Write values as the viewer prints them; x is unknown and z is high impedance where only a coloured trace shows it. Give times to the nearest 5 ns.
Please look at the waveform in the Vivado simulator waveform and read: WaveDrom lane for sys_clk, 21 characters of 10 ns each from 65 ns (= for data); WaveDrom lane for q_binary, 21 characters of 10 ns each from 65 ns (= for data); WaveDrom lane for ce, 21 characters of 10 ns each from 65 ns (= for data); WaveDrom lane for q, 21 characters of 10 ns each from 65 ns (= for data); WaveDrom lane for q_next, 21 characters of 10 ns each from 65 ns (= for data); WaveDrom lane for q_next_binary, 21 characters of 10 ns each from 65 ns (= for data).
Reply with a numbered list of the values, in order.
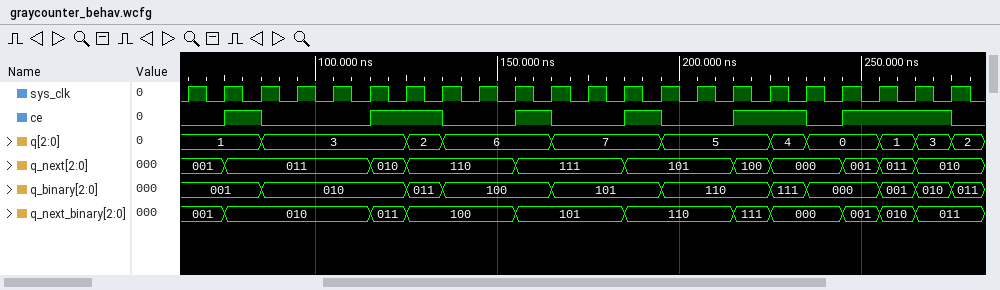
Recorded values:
1. {name: 'sys_clk', wave: 'p....................'}
2. {name: 'q_binary', wave: '=.=...==..=..=..==.==', data: '001 010 011 100 101 110 111 000 001 010'}
3. {name: 'ce', wave: '010..1.0.10.10.1.01..'}
4. {name: 'q', wave: '=.=...==..=..=..==.==', data: '1 3 2 6 7 5 4 0 1 3'}
5. {name: 'q_next', wave: '==...==..=..=..==.===', data: '001 011 010 110 111 101 100 000 001 011 010'}
6. {name: 'q_next_binary', wave: '==...==..=..=..==.===', data: '001 010 011 100 101 110 111 000 001 010 011'}
